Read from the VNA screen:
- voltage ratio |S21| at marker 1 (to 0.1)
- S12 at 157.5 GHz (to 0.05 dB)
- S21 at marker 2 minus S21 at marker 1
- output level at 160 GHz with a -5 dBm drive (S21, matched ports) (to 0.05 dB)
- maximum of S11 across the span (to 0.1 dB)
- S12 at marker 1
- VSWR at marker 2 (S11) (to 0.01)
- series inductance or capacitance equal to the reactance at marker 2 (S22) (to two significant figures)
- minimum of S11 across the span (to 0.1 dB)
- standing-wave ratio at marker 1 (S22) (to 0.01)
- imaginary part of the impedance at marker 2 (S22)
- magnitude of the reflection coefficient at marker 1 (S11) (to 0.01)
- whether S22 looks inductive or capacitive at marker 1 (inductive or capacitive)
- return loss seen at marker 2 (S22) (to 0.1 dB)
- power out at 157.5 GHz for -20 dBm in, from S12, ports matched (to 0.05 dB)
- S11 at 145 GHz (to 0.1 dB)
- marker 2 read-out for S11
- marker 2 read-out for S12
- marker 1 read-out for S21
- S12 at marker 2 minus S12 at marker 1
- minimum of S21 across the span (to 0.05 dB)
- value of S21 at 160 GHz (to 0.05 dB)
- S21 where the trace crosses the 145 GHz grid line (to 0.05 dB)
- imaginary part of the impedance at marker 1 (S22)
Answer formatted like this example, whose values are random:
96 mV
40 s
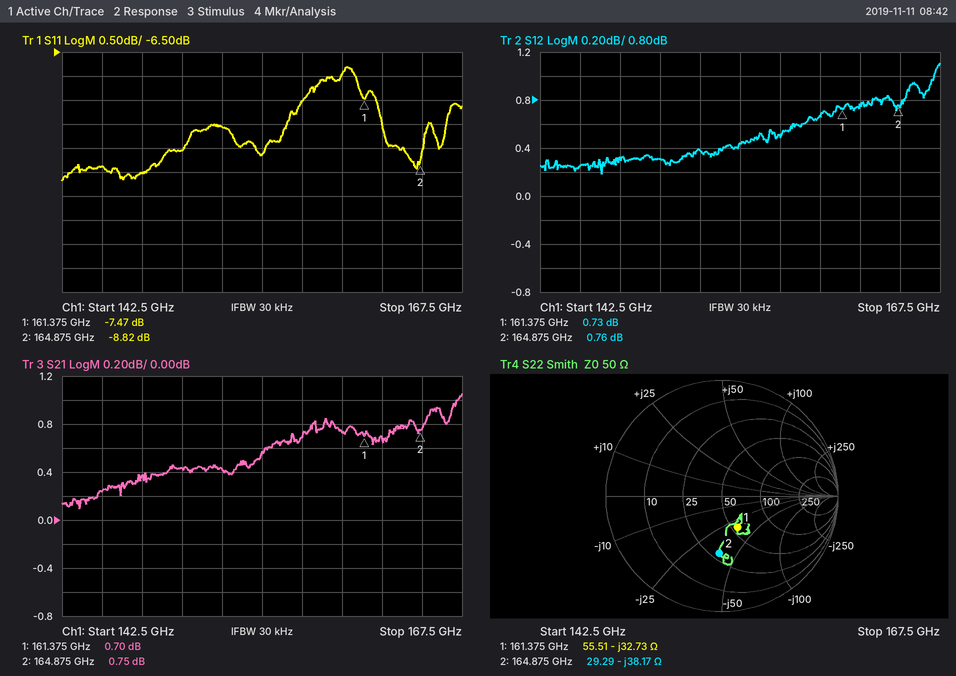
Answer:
1.1
0.50 dB
0.05 dB
-4.25 dBm
-6.8 dB
0.73 dB
2.14
25 fF
-9.2 dB
1.86
-38.17 Ω
0.42
capacitive
6.1 dB
-19.50 dBm
-8.9 dB
-8.82 dB
0.76 dB
0.70 dB
0.03 dB
0.10 dB
0.75 dB
0.25 dB
-32.73 Ω
